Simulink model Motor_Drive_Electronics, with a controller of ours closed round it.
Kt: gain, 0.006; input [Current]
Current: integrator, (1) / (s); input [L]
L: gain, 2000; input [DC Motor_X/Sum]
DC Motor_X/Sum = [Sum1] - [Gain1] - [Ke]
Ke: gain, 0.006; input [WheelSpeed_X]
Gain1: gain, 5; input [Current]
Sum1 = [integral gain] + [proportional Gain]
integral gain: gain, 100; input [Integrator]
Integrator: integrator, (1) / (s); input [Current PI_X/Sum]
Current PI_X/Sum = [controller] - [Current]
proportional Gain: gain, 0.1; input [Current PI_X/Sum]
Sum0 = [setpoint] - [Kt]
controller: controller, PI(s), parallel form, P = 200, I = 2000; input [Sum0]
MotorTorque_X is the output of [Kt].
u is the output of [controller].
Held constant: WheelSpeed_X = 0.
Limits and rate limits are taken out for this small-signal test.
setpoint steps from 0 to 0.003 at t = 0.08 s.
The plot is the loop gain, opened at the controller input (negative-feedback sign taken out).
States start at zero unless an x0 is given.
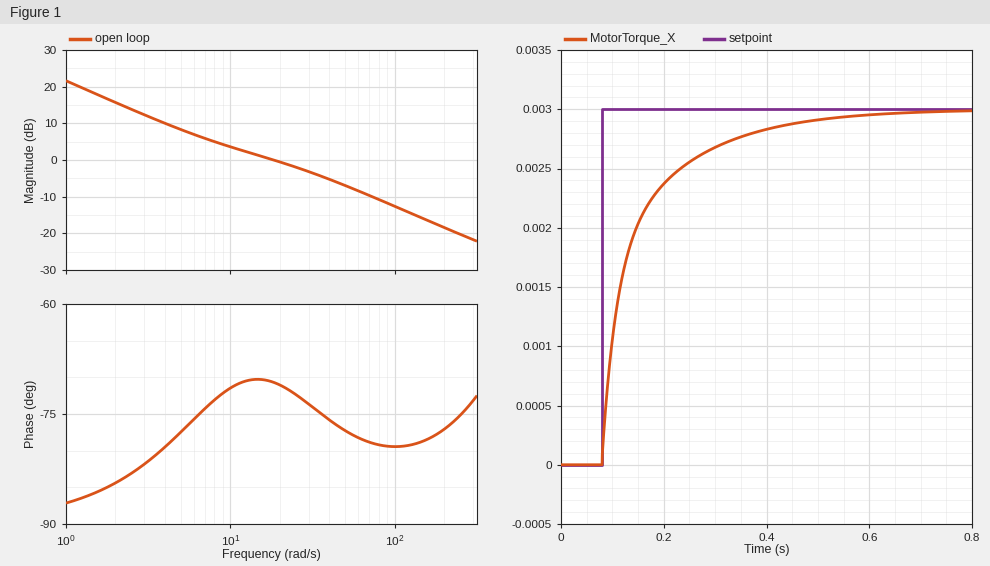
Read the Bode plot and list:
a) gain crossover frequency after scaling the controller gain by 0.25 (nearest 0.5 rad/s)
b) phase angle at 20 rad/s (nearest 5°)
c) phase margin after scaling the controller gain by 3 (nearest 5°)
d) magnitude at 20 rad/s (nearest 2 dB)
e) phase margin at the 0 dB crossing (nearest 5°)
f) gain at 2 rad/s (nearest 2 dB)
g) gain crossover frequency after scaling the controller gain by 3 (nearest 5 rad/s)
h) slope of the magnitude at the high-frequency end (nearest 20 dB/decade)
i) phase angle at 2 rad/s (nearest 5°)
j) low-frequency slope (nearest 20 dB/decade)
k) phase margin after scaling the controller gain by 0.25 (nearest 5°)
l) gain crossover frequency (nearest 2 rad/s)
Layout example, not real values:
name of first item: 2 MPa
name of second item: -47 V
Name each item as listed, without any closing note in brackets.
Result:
gain crossover frequency after scaling the controller gain by 0.25: 3.0 rad/s
phase angle at 20 rad/s: -70°
phase margin after scaling the controller gain by 3: 100°
magnitude at 20 rad/s: 0 dB
phase margin at the 0 dB crossing: 110°
gain at 2 rad/s: 16 dB
gain crossover frequency after scaling the controller gain by 3: 70 rad/s
slope of the magnitude at the high-frequency end: -20 dB/decade
phase angle at 2 rad/s: -85°
low-frequency slope: -20 dB/decade
phase margin after scaling the controller gain by 0.25: 100°
gain crossover frequency: 18 rad/s
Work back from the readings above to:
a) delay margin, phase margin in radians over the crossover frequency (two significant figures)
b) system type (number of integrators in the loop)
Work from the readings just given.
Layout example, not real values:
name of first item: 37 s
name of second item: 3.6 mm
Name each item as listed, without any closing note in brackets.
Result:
delay margin, phase margin in radians over the crossover frequency: 0.11 s
system type: 1
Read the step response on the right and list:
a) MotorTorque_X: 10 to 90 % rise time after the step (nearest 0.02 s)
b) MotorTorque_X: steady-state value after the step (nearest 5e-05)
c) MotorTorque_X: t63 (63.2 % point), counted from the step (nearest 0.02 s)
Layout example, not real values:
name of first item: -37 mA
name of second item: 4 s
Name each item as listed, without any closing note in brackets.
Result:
MotorTorque_X: 10 to 90 % rise time after the step: 0.22 s
MotorTorque_X: steady-state value after the step: 0.00300
MotorTorque_X: t63 (63.2 % point), counted from the step: 0.06 s
